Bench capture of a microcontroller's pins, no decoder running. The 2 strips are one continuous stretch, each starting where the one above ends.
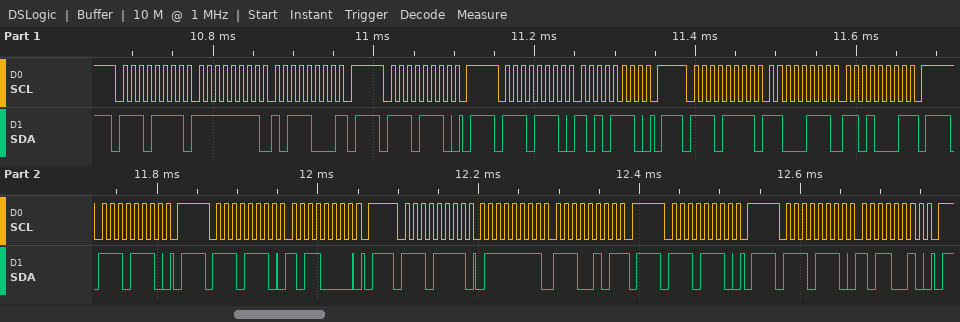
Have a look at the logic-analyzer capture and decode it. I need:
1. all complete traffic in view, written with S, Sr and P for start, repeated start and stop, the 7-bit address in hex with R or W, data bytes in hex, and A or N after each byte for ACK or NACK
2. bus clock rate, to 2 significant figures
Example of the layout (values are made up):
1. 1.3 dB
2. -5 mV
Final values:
1. S 77R A FF A B8 N P S 77W A P S 77W A AE A P S 77R A C7 A D1 N P S 77W A P S 77W A B0 A P S 77R A 7F A E5 N P S 77W A P S 77W A B2 A P
2. 100 kHz
